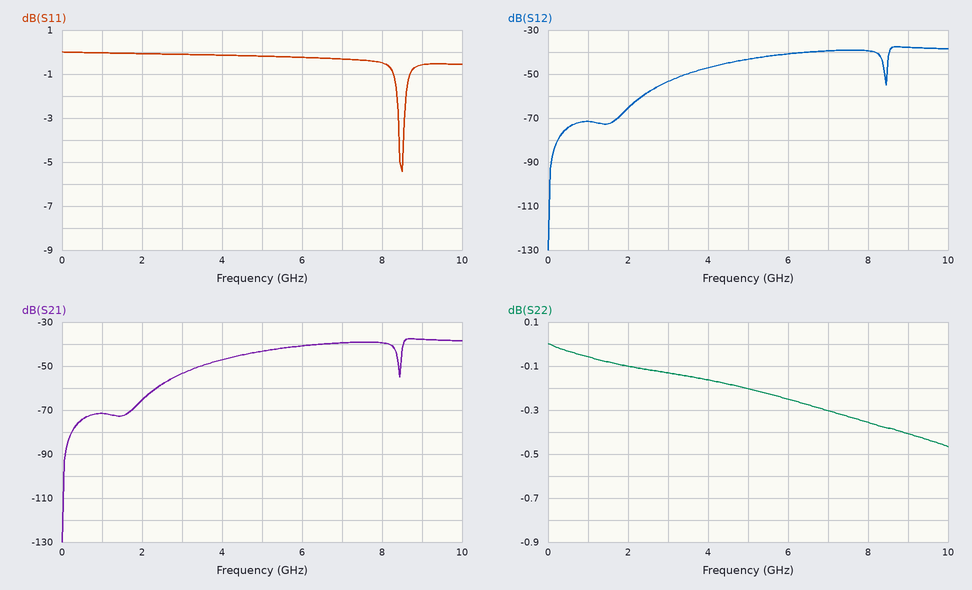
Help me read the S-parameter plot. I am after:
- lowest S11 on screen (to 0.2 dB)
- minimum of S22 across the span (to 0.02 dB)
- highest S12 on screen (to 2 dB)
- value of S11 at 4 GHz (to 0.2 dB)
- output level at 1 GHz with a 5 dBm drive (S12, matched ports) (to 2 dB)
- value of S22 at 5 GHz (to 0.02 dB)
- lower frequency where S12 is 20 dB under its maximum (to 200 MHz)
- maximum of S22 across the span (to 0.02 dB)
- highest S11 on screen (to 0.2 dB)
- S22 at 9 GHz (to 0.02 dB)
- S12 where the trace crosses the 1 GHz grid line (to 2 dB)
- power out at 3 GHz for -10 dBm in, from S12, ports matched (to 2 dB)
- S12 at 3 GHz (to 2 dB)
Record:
-5.4 dB
-0.46 dB
-38 dB
-0.2 dB
-66 dBm
-0.20 dB
2.6 GHz
0.00 dB
0.0 dB
-0.40 dB
-72 dB
-64 dBm
-54 dB
